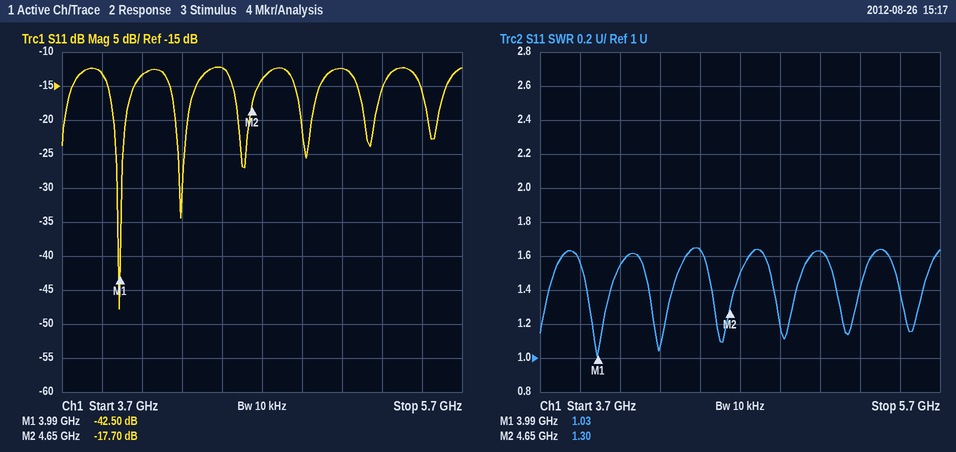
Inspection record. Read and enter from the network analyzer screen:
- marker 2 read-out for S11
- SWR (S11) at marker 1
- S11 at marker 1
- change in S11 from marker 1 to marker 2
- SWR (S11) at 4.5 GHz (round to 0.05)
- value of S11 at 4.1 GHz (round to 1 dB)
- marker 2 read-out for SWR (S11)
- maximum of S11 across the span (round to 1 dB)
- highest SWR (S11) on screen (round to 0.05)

-17.70 dB
1.03
-42.50 dB
24.80 dB
1.65
-13 dB
1.30
-12 dB
1.65
